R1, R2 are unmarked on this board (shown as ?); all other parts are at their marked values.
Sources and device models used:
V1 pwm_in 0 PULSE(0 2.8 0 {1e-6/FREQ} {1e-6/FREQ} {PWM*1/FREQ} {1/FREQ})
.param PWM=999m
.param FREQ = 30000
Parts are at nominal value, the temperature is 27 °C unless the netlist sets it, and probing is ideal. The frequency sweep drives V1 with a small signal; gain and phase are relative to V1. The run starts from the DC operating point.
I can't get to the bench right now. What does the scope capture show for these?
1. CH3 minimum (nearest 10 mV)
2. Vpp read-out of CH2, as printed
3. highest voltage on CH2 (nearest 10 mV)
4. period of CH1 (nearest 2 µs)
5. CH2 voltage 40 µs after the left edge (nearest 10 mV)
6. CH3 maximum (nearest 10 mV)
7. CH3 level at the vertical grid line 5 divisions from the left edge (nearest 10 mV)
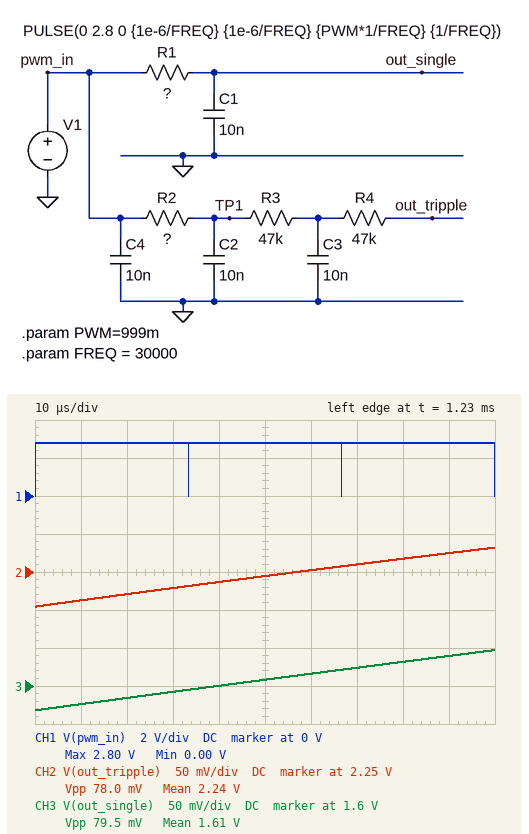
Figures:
1.57 V
78.0 mV
2.28 V
34 µs
2.24 V
1.65 V
1.61 V
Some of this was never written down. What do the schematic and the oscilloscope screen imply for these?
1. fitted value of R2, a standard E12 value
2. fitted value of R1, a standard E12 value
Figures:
18 kΩ
150 kΩ
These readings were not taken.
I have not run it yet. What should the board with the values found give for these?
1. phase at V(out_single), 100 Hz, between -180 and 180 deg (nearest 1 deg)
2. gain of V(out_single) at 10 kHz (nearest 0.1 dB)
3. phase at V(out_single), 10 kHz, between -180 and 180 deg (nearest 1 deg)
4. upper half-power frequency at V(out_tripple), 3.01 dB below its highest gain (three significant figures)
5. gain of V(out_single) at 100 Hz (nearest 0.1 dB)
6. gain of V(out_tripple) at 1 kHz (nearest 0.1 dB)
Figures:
-43 deg
-39.5 dB
-89 deg
218 Hz
-2.8 dB
-15.1 dB
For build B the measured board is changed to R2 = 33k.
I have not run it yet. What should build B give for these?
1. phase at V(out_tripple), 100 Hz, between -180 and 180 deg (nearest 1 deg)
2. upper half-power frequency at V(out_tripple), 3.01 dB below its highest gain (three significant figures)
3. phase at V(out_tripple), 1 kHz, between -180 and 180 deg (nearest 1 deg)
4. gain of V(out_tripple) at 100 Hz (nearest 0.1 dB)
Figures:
-37 deg
160 Hz
-126 deg
-1.4 dB
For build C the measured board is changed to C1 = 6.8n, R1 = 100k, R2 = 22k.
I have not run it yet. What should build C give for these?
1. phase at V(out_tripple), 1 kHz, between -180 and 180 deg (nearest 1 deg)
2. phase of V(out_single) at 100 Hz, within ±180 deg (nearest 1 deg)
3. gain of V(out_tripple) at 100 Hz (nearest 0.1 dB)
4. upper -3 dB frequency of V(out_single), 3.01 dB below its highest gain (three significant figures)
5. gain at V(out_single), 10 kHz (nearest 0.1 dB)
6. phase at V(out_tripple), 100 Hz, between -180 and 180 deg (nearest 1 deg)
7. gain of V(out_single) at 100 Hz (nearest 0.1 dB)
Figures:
-118 deg
-23 deg
-1.0 dB
234 Hz
-32.6 dB
-31 deg
-0.7 dB
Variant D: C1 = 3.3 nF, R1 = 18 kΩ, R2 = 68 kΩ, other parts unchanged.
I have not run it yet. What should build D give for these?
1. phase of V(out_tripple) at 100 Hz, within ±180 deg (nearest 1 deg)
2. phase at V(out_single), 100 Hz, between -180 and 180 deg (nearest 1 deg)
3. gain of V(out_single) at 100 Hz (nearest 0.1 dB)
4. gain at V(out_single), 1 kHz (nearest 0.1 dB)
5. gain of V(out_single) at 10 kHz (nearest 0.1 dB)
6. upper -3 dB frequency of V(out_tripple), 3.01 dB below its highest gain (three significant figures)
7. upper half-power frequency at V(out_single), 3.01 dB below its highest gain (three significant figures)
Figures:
-53 deg
-2 deg
0 dB
-0.6 dB
-11.7 dB
96.0 Hz
2.68 kHz
